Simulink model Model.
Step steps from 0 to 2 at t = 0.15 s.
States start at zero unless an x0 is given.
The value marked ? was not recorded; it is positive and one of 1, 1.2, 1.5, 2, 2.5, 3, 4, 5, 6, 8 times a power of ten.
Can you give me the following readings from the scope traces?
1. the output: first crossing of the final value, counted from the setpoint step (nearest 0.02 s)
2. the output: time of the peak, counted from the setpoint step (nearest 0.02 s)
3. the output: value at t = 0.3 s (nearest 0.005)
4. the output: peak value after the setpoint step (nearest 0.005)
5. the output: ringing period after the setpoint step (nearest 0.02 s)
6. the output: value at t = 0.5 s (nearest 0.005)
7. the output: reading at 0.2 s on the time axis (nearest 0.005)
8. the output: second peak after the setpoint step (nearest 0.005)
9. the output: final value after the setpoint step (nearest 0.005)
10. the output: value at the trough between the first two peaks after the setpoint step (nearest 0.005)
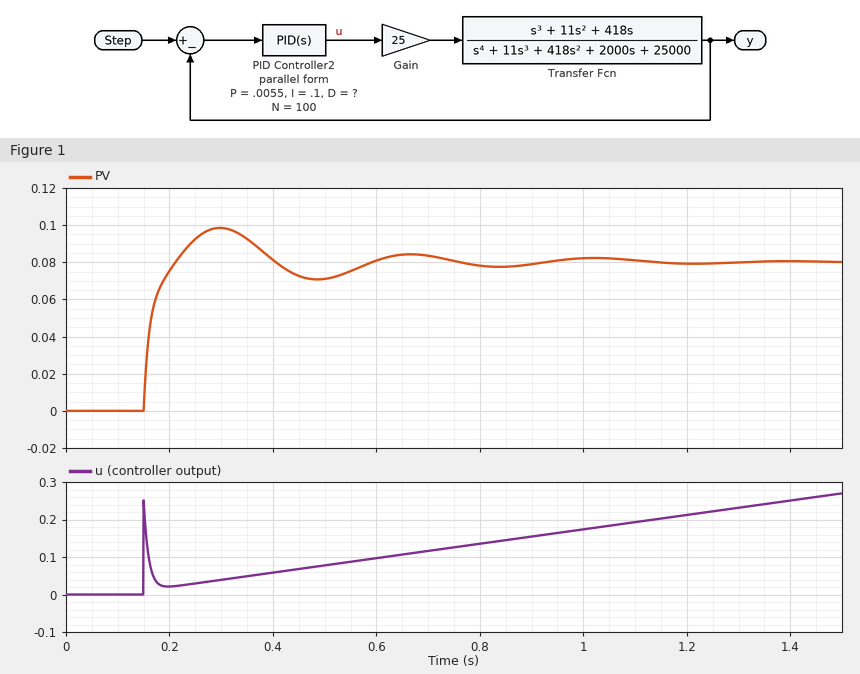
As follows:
0.06 s
0.14 s
0.100
0.100
0.36 s
0.070
0.075
0.085
0.080
0.070
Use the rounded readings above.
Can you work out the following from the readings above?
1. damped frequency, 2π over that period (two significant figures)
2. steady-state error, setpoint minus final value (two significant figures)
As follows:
17 rad/s
1.9
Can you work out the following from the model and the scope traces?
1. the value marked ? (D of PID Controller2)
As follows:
0.0012
